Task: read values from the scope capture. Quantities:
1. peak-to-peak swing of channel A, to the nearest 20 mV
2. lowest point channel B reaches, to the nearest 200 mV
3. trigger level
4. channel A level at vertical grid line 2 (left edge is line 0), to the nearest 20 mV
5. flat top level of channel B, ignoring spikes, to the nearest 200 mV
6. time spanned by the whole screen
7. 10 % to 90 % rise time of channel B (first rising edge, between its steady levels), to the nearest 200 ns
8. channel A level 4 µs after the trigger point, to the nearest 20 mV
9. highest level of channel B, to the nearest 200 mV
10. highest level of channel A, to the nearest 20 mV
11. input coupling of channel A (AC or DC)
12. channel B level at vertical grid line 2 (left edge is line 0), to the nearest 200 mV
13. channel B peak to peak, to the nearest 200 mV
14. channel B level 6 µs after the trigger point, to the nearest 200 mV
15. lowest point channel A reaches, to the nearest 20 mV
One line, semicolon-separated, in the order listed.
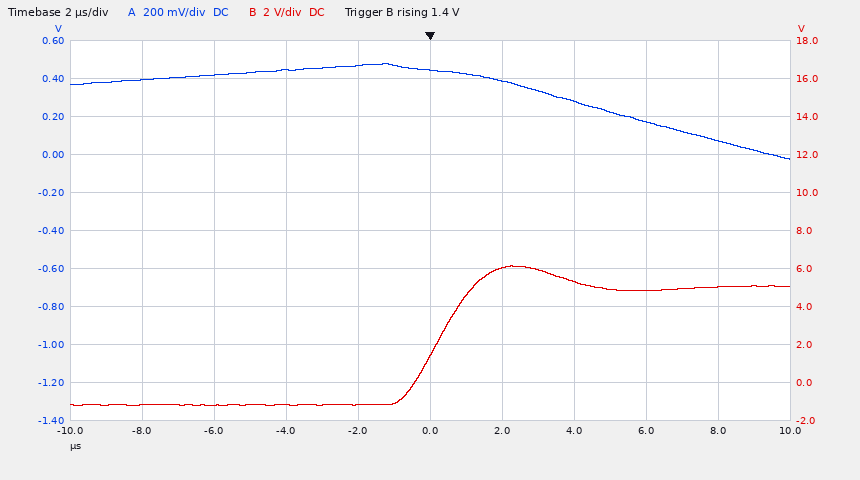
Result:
500 mV; -1.2 V; 1.4 V; 420 mV; 5.0 V; 20 µs; 1.6 µs; 280 mV; 6.2 V; 480 mV; DC; -1.2 V; 7.4 V; 4.8 V; -20 mV
